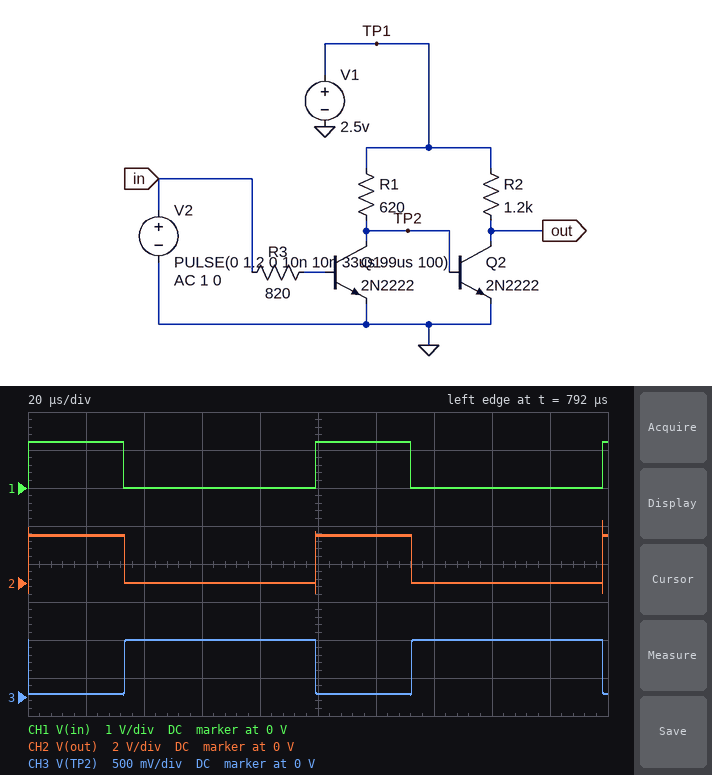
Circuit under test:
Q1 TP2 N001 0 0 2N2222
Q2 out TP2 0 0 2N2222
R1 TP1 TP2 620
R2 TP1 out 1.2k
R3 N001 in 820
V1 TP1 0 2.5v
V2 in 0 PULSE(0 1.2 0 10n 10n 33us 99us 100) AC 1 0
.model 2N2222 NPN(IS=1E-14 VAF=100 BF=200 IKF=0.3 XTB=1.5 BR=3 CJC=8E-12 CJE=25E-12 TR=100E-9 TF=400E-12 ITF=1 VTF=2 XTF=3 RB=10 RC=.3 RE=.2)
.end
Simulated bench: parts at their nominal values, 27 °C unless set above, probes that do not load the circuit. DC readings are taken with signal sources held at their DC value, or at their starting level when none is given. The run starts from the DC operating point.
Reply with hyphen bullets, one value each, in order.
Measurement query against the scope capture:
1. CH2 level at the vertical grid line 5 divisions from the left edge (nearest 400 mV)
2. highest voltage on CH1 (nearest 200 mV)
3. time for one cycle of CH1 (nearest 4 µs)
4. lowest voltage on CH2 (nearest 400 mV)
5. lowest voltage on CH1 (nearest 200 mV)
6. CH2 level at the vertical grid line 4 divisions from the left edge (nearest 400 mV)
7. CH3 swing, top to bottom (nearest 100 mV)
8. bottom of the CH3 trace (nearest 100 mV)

- 2.4 V
- 1.2 V
- 100 µs
- -400 mV
- 0 V
- 0 V
- 700 mV
- 0 V
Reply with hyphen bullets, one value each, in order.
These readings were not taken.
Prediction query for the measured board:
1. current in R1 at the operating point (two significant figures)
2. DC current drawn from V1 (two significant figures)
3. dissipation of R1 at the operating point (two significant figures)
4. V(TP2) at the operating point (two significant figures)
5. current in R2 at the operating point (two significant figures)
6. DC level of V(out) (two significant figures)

- 2.8 mA
- 4.9 mA
- 4.9 mW
- 750 mV
- 2.1 mA
- 14 mV
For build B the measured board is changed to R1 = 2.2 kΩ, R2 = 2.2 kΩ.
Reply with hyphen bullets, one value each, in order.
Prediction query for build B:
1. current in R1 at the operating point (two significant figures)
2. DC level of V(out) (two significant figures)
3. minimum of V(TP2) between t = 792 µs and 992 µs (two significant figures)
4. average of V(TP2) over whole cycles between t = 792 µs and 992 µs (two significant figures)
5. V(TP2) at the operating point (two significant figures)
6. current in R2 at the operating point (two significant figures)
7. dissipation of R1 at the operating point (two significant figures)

- 820 µA
- 16 mV
- 5.1 mV
- 470 mV
- 700 mV
- 1.1 mA
- 1.5 mW
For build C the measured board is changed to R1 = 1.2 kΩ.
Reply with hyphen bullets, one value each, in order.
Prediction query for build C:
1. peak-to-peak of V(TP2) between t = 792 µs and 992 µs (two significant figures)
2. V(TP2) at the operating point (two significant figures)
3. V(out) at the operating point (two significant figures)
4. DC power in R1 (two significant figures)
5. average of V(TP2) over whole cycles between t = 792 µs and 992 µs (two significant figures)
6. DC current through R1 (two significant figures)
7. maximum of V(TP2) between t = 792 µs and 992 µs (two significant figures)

- 710 mV
- 720 mV
- 17 mV
- 2.6 mW
- 490 mV
- 1.5 mA
- 730 mV
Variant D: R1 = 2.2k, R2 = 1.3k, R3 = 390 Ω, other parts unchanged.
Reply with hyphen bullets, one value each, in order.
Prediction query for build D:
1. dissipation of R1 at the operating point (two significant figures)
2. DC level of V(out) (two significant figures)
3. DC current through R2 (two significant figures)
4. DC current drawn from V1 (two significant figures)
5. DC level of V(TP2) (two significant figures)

- 1.5 mW
- 21 mV
- 1.9 mA
- 2.7 mA
- 710 mV
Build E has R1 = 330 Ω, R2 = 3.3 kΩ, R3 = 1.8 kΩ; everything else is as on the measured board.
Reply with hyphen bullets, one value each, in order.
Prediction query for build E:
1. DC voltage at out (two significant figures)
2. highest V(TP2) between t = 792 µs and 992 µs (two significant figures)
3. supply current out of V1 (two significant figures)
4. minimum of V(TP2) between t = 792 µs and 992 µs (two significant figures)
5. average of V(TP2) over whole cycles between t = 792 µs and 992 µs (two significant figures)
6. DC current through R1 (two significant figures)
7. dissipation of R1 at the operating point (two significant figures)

- 10 mV
- 790 mV
- 5.9 mA
- 68 mV
- 550 mV
- 5.2 mA
- 8.9 mW
